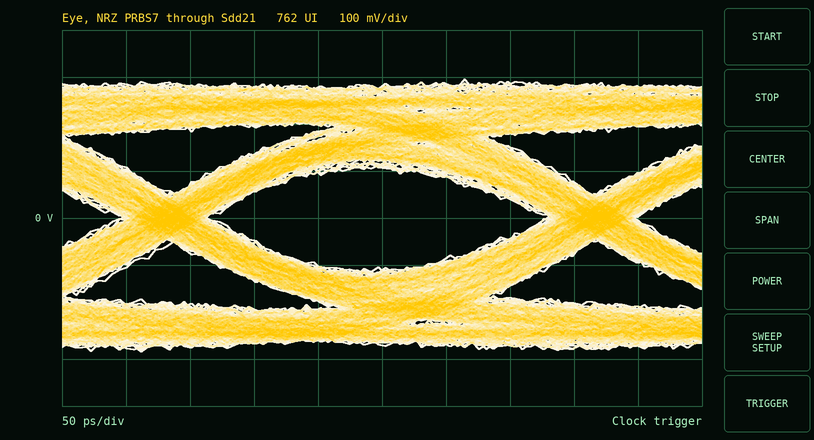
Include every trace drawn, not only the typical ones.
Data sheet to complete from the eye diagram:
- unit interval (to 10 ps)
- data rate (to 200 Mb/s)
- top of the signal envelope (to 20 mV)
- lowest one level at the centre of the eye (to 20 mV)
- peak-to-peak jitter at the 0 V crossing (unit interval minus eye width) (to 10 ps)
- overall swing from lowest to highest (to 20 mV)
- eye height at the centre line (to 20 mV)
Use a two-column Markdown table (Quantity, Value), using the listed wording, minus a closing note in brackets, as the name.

| Quantity | Value |
|---|---|
| unit interval | 330 ps |
| data rate | 3.0 Gb/s |
| top of the signal envelope | 300 mV |
| lowest one level at the centre of the eye | 100 mV |
| peak-to-peak jitter at the 0 V crossing (unit interval minus eye width) | 70 ps |
| overall swing from lowest to highest | 580 mV |
| eye height at the centre line | 220 mV |
